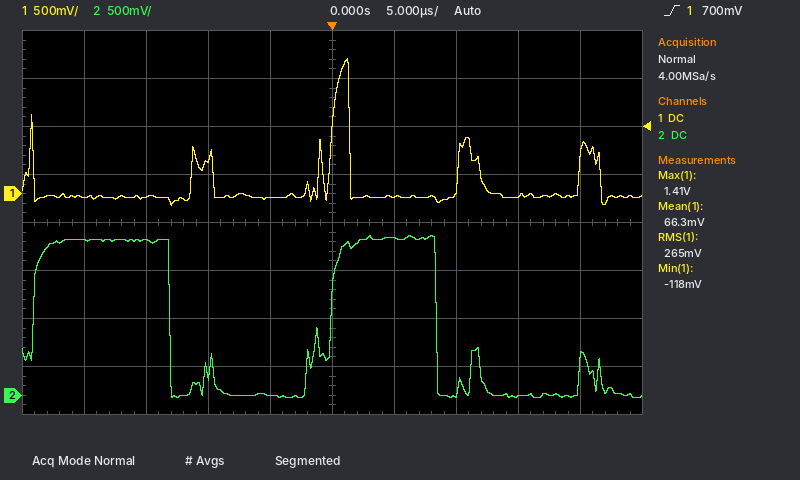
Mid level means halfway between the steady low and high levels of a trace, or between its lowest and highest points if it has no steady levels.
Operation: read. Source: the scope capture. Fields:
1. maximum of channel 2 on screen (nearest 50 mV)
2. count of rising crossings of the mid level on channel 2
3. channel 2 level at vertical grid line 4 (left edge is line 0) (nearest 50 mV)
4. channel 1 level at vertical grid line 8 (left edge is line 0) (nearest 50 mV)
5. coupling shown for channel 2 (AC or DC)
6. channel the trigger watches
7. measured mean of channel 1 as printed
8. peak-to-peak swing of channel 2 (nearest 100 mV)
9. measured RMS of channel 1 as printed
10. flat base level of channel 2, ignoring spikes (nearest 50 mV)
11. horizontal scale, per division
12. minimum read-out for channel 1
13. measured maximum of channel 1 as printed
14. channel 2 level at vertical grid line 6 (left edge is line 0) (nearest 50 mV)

1.65 V
2
0 mV
0 mV
DC
channel 1
66.3 mV
1.70 V
265 mV
0 mV
5 µs
-118 mV
1.41 V
1.65 V
